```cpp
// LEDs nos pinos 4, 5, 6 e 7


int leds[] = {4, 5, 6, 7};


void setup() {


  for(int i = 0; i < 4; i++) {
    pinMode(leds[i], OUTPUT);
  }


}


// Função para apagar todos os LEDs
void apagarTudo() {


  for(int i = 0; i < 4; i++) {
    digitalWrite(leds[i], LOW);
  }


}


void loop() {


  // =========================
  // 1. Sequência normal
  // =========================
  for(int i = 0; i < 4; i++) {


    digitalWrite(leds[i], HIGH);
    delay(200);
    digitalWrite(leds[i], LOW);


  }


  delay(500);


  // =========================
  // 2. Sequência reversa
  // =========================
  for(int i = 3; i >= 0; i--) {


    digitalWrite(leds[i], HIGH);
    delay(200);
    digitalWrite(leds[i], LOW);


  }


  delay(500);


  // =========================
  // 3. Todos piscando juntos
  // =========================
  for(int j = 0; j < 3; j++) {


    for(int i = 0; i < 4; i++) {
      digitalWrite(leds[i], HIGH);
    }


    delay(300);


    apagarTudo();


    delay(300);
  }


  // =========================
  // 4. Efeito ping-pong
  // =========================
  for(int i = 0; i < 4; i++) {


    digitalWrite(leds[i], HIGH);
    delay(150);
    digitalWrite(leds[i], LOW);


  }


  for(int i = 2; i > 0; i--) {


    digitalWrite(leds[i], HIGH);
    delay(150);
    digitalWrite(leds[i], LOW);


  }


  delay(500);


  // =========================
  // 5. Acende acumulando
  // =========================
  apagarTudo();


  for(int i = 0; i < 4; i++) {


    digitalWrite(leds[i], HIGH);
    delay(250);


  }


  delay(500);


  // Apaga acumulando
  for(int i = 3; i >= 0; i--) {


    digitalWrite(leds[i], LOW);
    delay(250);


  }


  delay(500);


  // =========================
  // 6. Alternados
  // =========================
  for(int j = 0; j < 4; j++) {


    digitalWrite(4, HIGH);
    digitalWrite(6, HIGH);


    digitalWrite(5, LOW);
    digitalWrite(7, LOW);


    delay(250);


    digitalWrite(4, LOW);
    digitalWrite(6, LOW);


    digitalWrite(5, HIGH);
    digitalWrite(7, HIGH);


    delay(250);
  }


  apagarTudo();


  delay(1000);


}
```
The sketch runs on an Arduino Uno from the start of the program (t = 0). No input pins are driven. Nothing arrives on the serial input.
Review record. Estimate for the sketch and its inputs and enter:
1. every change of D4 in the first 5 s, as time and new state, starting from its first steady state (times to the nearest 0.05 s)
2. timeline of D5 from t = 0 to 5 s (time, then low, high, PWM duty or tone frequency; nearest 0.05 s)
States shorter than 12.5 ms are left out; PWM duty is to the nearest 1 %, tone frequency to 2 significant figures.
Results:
0 s high; 0.2 s low; 1.9 s high; 2.1 s low; 2.6 s high; 2.9 s low; 3.2 s high; 3.5 s low; 3.8 s high; 4.1 s low; 4.4 s high; 4.55 s low
0 s low; 0.2 s high; 0.4 s low; 1.7 s high; 1.9 s low; 2.6 s high; 2.9 s low; 3.2 s high; 3.5 s low; 3.8 s high; 4.1 s low; 4.55 s high; 4.7 s low
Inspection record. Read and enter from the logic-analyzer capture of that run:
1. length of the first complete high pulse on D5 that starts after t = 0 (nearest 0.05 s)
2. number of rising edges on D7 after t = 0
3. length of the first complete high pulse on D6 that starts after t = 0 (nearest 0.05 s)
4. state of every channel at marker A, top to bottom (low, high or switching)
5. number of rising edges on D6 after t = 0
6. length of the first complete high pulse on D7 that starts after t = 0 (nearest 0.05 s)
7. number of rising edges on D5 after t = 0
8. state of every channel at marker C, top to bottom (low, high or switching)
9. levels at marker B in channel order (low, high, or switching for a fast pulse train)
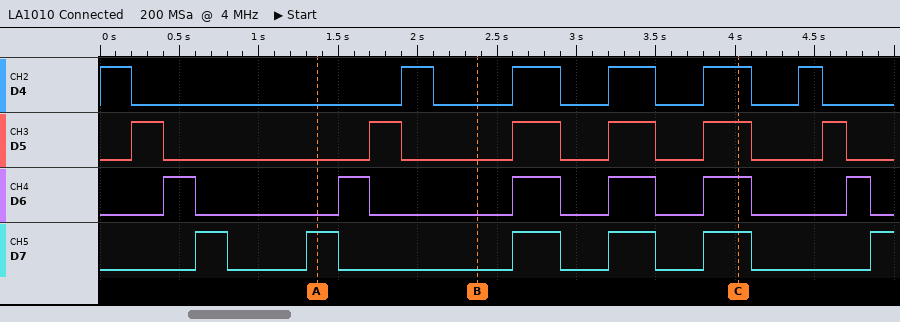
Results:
0.20 s
6
0.20 s
D4 low, D5 low, D6 low, D7 high
6
0.20 s
6
D4 high, D5 high, D6 high, D7 high
D4 low, D5 low, D6 low, D7 low
